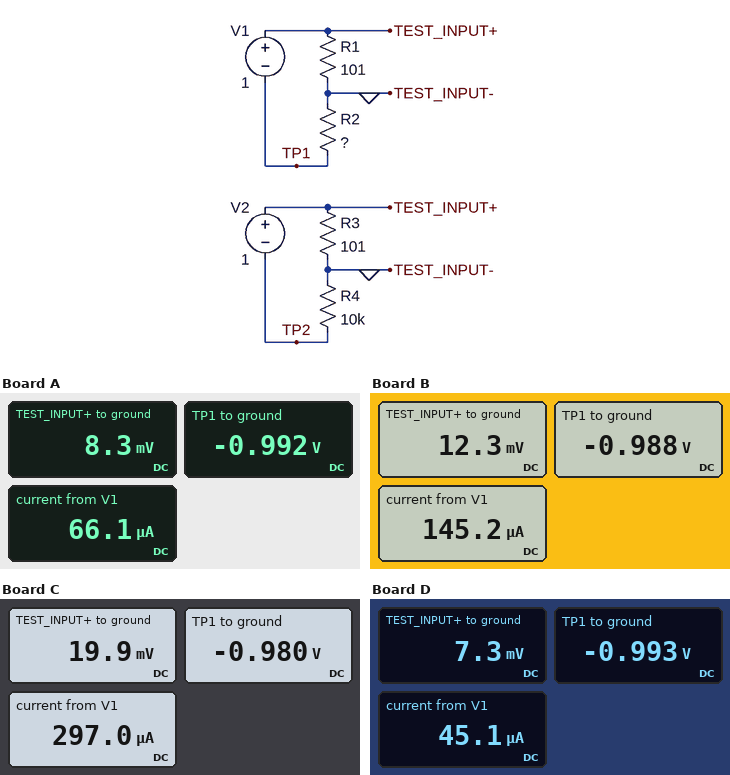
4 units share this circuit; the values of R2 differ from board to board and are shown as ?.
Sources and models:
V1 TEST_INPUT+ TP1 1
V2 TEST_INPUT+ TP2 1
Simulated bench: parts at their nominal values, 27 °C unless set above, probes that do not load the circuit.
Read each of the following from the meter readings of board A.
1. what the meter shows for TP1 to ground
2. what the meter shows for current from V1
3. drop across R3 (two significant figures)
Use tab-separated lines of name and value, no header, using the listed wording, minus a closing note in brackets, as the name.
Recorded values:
what the meter shows for TP1 to ground	-0.992 V
what the meter shows for current from V1	66.1 µA
drop across R3	8.3 mV
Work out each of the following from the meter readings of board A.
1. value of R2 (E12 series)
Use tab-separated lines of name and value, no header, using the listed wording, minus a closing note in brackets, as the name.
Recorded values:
value of R2	15 kΩ
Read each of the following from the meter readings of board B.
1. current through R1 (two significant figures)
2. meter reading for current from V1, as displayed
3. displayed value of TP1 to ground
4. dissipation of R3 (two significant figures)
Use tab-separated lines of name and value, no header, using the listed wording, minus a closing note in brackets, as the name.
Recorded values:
current through R1	120 µA
meter reading for current from V1, as displayed	145.2 µA
displayed value of TP1 to ground	-0.988 V
dissipation of R3	1.5 µW
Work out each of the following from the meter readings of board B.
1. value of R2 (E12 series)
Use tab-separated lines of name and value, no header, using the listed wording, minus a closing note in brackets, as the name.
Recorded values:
value of R2	6.8 kΩ
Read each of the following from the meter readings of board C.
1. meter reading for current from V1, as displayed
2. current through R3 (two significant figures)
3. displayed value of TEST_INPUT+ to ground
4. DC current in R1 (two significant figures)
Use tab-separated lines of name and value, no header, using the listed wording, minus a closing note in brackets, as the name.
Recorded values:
meter reading for current from V1, as displayed	297.0 µA
current through R3	200 µA
displayed value of TEST_INPUT+ to ground	19.9 mV
DC current in R1	200 µA
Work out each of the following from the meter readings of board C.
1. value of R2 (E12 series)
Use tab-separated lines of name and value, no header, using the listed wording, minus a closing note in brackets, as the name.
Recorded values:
value of R2	3.3 kΩ
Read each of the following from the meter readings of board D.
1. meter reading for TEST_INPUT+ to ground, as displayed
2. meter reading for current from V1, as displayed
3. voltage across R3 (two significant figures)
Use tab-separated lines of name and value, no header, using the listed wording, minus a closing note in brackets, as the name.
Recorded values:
meter reading for TEST_INPUT+ to ground, as displayed	7.3 mV
meter reading for current from V1, as displayed	45.1 µA
voltage across R3	7.3 mV
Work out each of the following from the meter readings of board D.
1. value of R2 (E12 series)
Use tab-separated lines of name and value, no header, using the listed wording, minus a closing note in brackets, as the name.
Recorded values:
value of R2	22 kΩ
